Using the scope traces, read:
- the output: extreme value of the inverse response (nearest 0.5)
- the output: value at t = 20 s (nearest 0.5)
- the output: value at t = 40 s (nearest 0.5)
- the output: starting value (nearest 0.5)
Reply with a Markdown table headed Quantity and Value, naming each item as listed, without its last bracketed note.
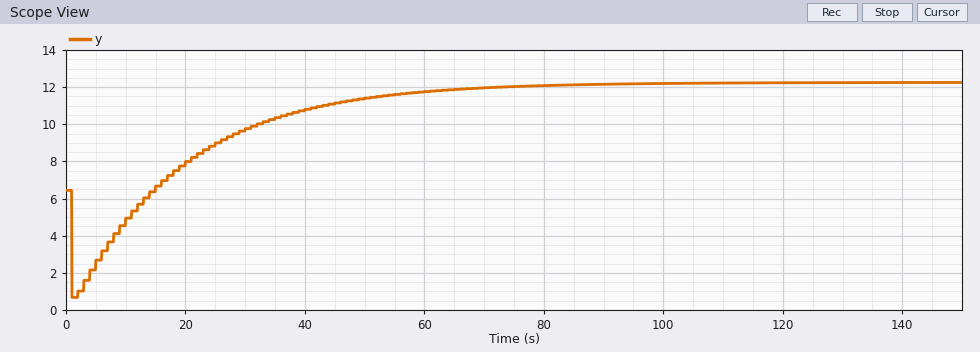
| Quantity | Value |
|---|---|
| the output: extreme value of the inverse response | 0.5 |
| the output: value at t = 20 s | 8.0 |
| the output: value at t = 40 s | 11.0 |
| the output: starting value | 6.5 |
